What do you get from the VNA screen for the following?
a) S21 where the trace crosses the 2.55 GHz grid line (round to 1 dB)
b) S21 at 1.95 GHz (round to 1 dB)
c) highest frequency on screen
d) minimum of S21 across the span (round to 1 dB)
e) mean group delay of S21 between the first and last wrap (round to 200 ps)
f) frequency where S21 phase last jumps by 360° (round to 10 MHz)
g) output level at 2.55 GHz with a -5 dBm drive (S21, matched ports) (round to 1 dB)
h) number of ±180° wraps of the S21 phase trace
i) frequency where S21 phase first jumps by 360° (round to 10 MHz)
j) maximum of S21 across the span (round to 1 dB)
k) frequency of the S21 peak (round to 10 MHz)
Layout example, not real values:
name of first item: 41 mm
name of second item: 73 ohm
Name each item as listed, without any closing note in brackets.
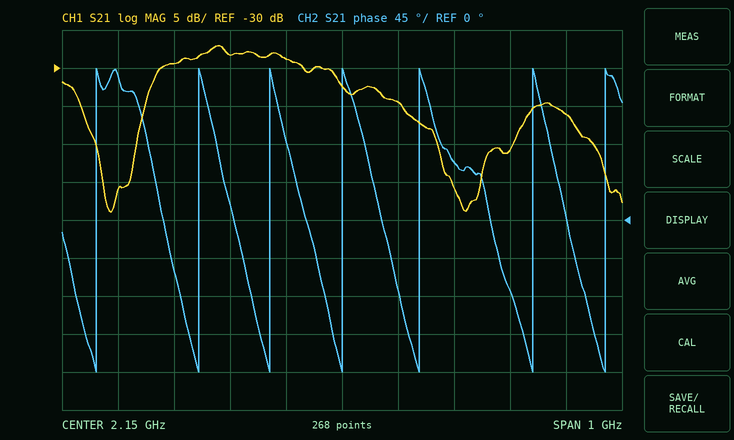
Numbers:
S21 where the trace crosses the 2.55 GHz grid line: -36 dB
S21 at 1.95 GHz: -28 dB
highest frequency on screen: 2.65 GHz
minimum of S21 across the span: -49 dB
mean group delay of S21 between the first and last wrap: 6.6 ns
frequency where S21 phase last jumps by 360°: 2.62 GHz
output level at 2.55 GHz with a -5 dBm drive (S21, matched ports): -41 dBm
number of ±180° wraps of the S21 phase trace: 7
frequency where S21 phase first jumps by 360°: 1.71 GHz
maximum of S21 across the span: -27 dB
frequency of the S21 peak: 1.93 GHz
